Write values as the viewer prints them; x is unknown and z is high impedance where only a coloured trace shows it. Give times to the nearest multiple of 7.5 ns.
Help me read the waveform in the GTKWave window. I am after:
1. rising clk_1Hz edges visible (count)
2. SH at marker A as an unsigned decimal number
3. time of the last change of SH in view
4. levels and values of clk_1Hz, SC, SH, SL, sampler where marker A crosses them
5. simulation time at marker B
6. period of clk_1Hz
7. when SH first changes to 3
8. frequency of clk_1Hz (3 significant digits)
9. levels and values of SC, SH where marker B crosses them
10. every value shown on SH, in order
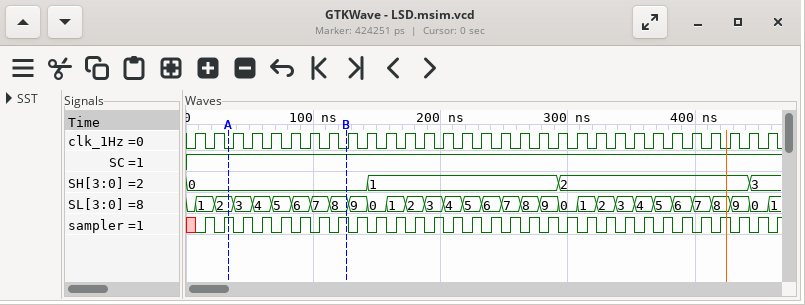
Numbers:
31
0
442.5 ns
clk_1Hz=0, SC=1, SH=0, SL=2, sampler=1
127.5 ns
15 ns
442.5 ns
66.7 MHz
SC=1, SH=0
0, 1, 2, 3
